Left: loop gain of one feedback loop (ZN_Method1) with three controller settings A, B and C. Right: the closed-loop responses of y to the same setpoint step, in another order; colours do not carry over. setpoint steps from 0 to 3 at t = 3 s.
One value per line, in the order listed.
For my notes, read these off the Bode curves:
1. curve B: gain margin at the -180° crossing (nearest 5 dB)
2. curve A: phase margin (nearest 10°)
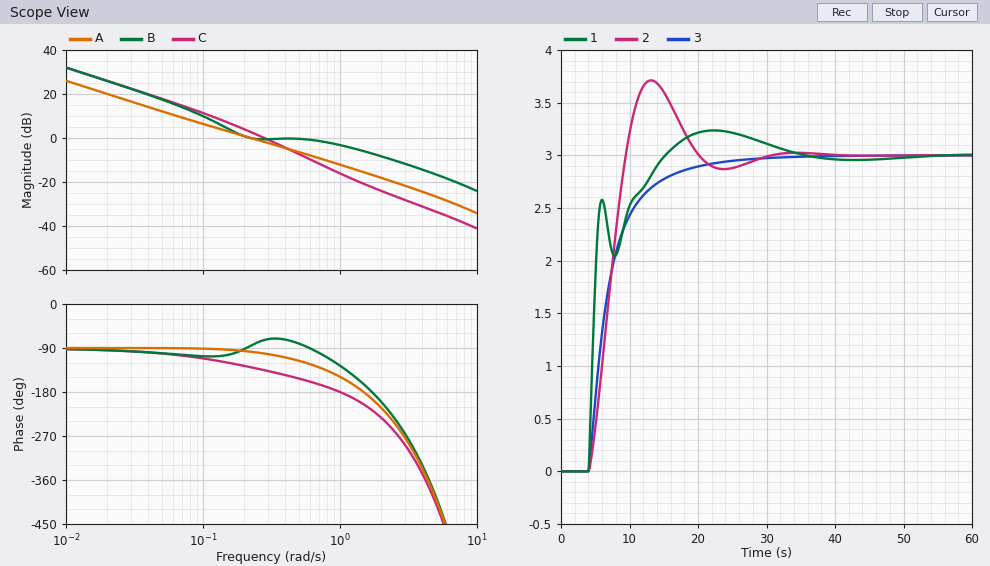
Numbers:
5 dB
80°
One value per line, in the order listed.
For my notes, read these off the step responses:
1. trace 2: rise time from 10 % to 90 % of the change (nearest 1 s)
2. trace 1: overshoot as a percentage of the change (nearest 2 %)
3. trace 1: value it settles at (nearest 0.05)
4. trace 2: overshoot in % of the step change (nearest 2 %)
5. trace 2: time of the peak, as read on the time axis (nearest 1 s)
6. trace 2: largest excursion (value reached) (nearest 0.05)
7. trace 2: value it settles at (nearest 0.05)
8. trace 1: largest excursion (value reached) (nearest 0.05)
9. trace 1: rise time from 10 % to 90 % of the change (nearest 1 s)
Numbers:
4 s
8 %
3.00
24 %
13 s
3.70
3.00
3.25
8 s
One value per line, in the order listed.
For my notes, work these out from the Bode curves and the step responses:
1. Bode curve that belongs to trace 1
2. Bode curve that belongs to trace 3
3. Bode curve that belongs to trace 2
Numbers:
B
A
C
